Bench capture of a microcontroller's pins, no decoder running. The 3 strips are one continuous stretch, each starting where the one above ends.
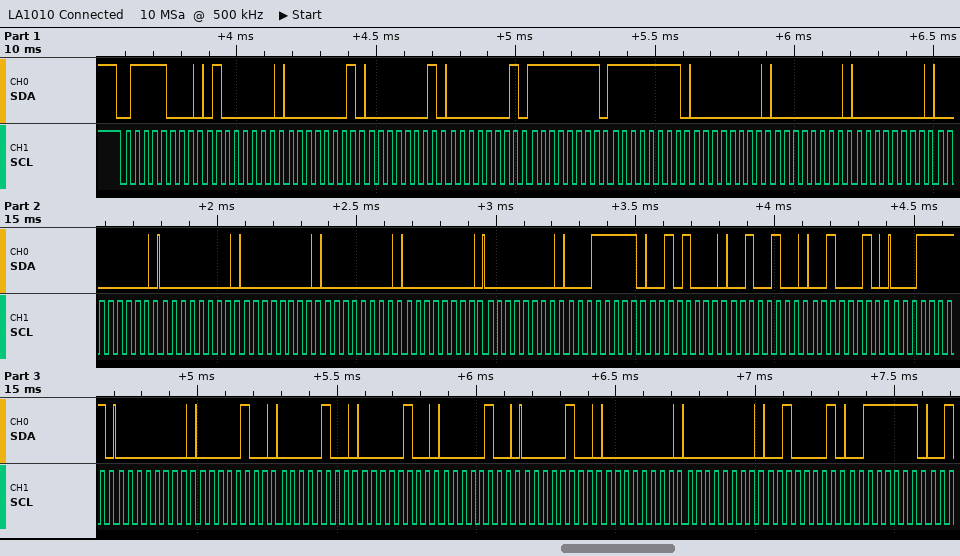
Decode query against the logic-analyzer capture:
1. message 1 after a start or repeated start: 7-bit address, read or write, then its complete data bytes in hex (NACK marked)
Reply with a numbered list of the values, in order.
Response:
1. 0x3C write: 40 01 01 01 FF FF 00 00 00 00 00 00 00 00 00 1F 28 24 22 1F 00 04 04 04 04 04 00 00 21 3F
